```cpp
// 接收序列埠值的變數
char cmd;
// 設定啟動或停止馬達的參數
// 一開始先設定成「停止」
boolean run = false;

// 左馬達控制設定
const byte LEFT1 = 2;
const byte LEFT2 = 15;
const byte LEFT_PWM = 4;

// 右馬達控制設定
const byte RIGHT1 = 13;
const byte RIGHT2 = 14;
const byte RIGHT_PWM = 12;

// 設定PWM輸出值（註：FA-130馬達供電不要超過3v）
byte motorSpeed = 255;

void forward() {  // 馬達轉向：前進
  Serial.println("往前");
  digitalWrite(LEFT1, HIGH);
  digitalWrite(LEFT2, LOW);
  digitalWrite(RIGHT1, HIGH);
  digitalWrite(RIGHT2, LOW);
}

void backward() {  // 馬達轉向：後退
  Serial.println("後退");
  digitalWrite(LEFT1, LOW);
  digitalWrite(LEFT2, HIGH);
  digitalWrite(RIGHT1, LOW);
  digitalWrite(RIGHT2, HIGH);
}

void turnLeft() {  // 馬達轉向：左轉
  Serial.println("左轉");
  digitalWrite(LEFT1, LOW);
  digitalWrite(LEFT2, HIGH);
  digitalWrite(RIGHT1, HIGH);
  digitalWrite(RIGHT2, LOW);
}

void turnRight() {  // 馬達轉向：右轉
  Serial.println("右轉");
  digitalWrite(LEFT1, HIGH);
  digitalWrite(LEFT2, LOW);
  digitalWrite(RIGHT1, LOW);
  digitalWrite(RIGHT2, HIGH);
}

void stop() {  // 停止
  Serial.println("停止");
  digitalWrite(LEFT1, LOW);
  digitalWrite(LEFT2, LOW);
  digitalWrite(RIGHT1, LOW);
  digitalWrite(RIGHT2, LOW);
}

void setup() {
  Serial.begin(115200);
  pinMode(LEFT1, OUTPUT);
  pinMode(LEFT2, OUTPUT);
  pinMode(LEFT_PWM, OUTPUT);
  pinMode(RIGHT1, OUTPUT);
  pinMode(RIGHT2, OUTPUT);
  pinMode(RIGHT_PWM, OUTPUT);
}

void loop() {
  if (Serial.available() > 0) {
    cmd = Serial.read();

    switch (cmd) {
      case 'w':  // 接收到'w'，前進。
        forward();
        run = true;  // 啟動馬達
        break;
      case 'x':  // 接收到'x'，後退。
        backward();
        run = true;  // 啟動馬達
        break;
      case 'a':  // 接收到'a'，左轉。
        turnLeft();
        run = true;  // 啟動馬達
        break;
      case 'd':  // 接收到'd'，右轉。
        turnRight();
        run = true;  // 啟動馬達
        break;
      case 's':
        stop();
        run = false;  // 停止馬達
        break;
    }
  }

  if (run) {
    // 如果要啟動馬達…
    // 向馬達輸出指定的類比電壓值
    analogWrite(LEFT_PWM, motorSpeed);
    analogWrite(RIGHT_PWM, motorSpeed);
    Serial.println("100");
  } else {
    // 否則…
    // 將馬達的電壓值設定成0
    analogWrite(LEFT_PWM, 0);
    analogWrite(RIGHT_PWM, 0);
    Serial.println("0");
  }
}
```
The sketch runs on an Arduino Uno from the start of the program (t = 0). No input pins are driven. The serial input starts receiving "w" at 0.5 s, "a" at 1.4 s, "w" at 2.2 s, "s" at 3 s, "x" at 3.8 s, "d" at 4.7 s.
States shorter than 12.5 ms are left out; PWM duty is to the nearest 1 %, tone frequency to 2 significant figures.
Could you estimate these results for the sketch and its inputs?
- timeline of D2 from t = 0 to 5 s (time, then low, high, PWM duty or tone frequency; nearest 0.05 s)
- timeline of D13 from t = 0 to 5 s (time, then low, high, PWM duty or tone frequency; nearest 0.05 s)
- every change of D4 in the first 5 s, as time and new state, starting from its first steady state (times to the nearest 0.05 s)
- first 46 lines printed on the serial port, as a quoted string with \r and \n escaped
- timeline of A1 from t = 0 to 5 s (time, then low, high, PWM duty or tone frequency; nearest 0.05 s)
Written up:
0 s low; 0.5 s high; 1.4 s low; 2.2 s high; 3 s low; 4.7 s high
0 s low; 0.5 s high; 3 s low
0 s low; 0.5 s high; 3 s low; 3.8 s high
"0\r\n0\r\n0\r\n0\r\n0\r\n0\r\n0\r\n0\r\n0\r\n0\r\n0\r\n0\r\n0\r\n0\r\n0\r\n0\r\n0\r\n0\r\n0\r\n0\r\n0\r\n0\r\n0\r\n0\r\n0\r\n0\r\n0\r\n0\r\n0\r\n0\r\n0\r\n0\r\n0\r\n0\r\n0\r\n0\r\n0\r\n0\r\n0\r\n0\r\n0\r\n0\r\n0\r\n0\r\n0\r\n0\r\n"
0 s low; 1.4 s high; 2.2 s low; 3.8 s high; 4.7 s low
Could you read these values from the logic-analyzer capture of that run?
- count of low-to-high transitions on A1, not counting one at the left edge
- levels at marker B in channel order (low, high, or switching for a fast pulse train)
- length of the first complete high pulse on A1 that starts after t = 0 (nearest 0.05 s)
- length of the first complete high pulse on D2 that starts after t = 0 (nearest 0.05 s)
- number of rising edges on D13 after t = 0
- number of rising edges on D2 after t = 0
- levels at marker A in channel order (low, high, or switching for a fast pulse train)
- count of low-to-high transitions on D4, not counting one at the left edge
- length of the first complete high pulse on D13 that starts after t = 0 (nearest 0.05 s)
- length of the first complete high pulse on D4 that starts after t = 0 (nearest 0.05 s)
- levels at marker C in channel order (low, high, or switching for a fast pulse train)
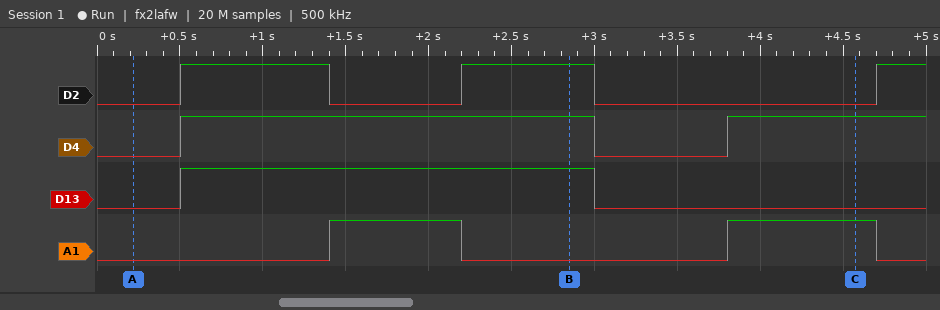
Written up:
2
D2 high, D4 high, D13 high, A1 low
0.80 s
0.90 s
1
3
D2 low, D4 low, D13 low, A1 low
2
2.50 s
2.50 s
D2 low, D4 high, D13 low, A1 high
